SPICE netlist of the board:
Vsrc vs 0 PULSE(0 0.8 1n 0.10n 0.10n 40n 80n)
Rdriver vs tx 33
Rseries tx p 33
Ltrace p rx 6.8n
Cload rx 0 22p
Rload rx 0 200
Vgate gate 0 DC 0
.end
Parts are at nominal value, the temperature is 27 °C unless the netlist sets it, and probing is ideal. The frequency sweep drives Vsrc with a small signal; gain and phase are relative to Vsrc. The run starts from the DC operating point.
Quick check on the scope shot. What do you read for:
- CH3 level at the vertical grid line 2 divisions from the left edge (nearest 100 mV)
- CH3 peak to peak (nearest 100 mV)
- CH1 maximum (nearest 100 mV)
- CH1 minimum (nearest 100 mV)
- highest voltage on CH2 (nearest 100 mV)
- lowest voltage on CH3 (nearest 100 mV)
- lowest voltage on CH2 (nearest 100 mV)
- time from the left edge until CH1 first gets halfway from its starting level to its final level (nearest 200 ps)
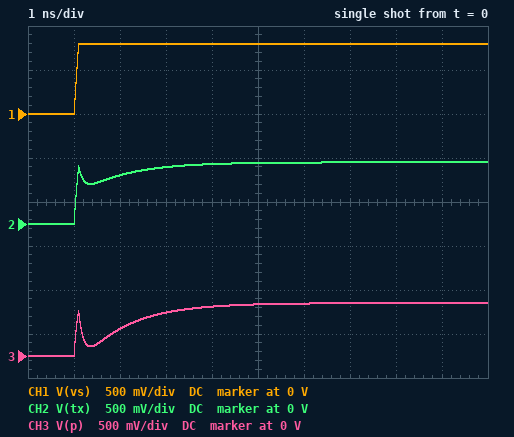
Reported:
300 mV
600 mV
800 mV
0 V
700 mV
0 V
0 V
1.0 ns
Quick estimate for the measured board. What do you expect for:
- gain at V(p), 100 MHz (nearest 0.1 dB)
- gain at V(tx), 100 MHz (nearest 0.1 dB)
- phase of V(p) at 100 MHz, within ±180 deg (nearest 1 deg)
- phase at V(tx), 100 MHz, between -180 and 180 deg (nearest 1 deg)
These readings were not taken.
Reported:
-4.5 dB
-2.3 dB
-35 deg
-13 deg
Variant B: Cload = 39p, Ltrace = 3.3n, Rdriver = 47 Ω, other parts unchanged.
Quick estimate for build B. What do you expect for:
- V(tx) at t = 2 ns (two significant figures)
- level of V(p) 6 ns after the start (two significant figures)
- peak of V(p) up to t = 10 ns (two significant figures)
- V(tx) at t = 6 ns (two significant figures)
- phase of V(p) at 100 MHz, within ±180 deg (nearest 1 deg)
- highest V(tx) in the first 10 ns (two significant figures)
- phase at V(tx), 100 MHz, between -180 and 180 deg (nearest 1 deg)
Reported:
440 mV
510 mV
560 mV
630 mV
-55 deg
660 mV
-19 deg
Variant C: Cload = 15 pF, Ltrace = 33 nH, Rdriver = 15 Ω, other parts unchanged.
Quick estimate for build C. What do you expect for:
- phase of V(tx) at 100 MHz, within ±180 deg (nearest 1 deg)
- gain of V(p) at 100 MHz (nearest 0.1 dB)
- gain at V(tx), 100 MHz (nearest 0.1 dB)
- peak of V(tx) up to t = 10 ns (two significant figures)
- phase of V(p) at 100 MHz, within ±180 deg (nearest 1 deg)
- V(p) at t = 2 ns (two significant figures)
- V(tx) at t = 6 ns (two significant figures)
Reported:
-5 deg
-3.3 dB
-1.0 dB
780 mV
-21 deg
350 mV
750 mV
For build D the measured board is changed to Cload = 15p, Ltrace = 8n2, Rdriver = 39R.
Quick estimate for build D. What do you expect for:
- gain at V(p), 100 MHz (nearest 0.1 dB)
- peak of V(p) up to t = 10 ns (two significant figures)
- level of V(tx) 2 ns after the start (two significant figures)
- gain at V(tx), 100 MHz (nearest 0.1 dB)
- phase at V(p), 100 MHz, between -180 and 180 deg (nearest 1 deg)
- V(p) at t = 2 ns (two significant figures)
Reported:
-3.9 dB
590 mV
570 mV
-2.1 dB
-27 deg
370 mV
